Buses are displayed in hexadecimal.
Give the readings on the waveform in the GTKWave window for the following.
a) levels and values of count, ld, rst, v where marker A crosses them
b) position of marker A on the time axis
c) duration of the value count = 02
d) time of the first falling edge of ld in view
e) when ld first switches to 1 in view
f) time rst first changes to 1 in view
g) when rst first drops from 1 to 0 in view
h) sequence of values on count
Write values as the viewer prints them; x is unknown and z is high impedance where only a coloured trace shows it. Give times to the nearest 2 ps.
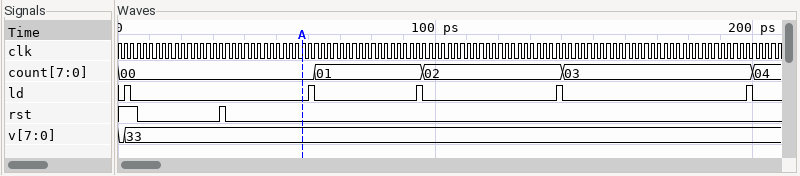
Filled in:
count=00, ld=0, rst=0, v=33
58 ps
44 ps
4 ps
2 ps
32 ps
6 ps
00, 01, 02, 03, 04
